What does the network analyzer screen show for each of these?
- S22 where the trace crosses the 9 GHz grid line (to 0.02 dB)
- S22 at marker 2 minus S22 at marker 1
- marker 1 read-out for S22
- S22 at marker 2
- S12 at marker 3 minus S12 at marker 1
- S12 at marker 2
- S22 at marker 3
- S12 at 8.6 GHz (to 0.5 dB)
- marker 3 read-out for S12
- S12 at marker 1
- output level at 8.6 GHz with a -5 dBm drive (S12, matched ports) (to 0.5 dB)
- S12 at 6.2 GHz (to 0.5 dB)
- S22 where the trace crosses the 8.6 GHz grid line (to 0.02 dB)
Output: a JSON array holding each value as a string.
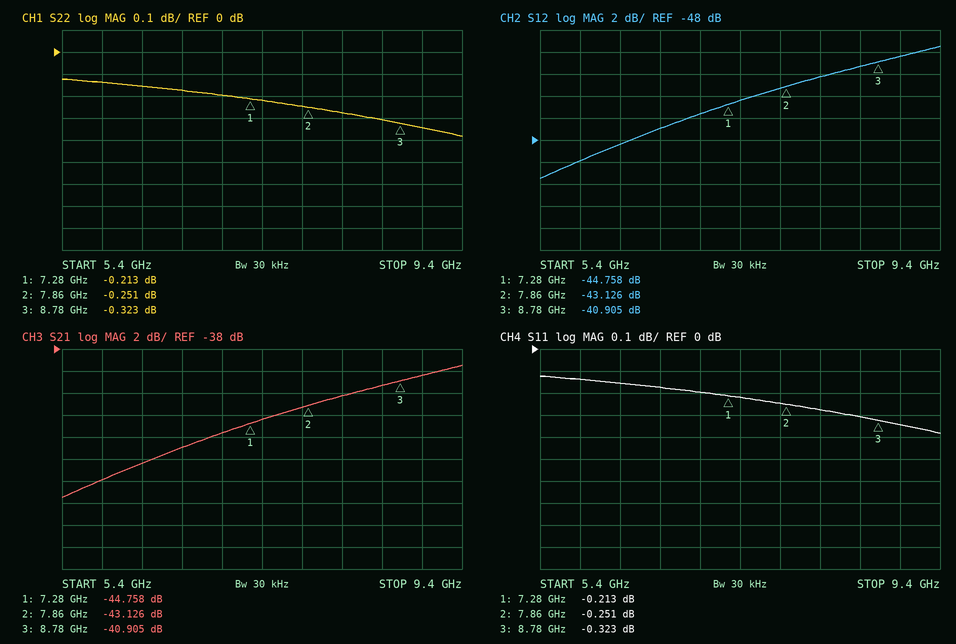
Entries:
["-0.34 dB", "-0.038 dB", "-0.213 dB", "-0.251 dB", "3.853 dB", "-43.126 dB", "-0.323 dB", "-41.5 dB", "-40.905 dB", "-44.758 dB", "-46.5 dBm", "-48.5 dB", "-0.30 dB"]
